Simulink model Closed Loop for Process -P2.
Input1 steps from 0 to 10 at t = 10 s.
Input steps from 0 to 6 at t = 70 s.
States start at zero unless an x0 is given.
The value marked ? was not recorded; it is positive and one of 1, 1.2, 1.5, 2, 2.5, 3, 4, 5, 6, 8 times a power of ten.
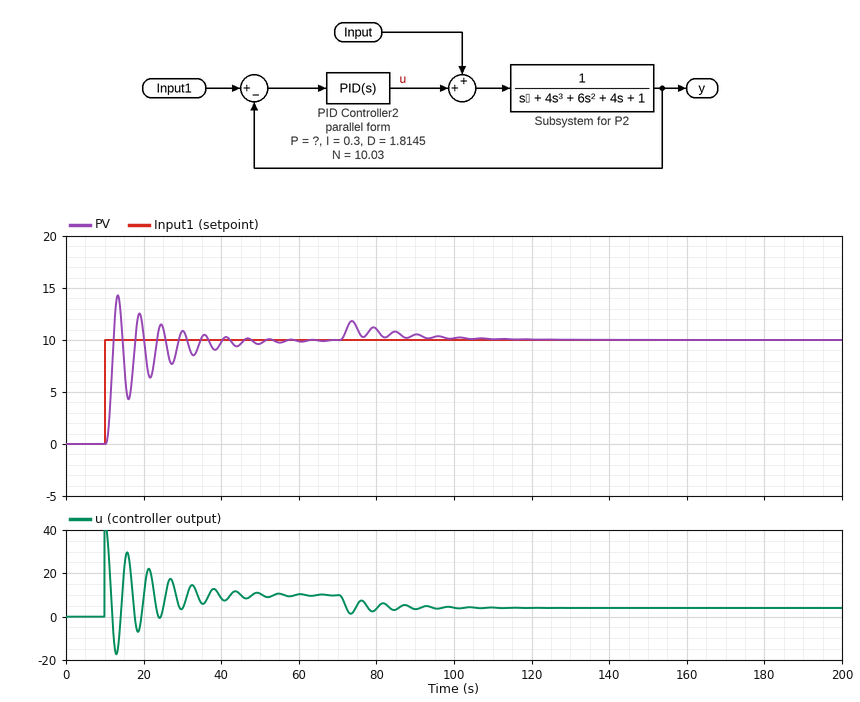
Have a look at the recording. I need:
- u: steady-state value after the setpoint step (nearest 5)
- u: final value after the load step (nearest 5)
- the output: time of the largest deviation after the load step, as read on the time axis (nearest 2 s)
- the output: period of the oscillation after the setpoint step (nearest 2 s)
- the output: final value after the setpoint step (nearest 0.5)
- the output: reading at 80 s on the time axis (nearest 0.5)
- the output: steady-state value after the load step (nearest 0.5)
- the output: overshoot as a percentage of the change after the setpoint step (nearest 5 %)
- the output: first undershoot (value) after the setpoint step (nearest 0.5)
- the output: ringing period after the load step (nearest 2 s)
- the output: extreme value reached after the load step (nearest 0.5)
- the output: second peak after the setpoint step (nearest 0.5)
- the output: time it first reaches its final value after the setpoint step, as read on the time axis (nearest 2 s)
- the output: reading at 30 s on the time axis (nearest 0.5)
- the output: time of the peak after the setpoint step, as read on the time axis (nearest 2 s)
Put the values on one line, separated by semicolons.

10; 5; 74 s; 6 s; 10.0; 11.0; 10.0; 45 %; 4.5; 6 s; 12.0; 12.5; 12 s; 11.0; 14 s
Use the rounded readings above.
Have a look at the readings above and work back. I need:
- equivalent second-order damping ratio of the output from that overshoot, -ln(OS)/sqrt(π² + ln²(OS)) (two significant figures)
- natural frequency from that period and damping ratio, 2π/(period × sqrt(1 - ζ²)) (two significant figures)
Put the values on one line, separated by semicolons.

0.25; 1.1 rad/s
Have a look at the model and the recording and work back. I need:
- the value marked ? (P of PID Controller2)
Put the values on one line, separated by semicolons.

4
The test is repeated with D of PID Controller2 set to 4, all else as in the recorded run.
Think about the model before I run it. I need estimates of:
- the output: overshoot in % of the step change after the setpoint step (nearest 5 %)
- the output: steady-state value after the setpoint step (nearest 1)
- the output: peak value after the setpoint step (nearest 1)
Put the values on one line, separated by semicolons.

35 %; 10; 14
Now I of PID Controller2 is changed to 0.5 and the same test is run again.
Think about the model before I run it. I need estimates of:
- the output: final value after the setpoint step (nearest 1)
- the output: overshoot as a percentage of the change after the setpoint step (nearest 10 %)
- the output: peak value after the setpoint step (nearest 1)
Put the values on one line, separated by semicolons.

10; 50 %; 15
